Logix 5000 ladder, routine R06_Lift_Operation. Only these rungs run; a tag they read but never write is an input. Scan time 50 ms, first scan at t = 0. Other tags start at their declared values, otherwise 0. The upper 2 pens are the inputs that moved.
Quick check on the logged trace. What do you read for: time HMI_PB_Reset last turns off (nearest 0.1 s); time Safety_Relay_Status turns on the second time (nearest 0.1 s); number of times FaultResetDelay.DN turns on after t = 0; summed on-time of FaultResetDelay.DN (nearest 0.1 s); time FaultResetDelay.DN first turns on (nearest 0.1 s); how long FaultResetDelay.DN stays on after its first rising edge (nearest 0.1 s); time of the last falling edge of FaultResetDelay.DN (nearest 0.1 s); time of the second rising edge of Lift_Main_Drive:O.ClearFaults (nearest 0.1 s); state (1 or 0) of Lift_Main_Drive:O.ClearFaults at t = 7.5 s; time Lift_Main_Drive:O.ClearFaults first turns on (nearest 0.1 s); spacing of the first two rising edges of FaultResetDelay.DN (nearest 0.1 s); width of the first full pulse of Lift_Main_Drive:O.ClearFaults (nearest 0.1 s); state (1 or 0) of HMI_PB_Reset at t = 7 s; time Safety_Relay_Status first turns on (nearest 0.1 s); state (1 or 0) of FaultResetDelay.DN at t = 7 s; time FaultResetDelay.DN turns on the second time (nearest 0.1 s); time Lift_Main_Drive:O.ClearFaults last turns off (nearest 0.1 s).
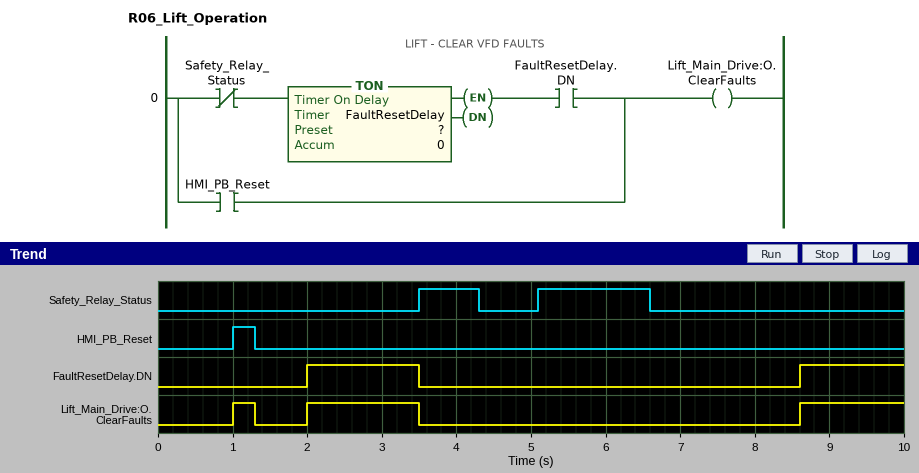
1.3 s
5.1 s
2
2.9 s
2.0 s
1.5 s
3.5 s
2.0 s
0
1.0 s
6.6 s
0.3 s
0
3.5 s
0
8.6 s
3.5 s
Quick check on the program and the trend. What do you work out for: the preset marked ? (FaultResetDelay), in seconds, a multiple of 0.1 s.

2.0 s
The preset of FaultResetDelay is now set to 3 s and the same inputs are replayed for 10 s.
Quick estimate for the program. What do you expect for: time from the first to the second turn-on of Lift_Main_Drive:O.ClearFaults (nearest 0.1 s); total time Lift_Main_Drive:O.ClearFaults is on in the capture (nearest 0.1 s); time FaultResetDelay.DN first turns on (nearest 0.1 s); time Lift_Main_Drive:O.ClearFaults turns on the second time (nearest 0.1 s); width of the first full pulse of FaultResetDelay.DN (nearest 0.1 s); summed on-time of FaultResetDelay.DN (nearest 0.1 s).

2.0 s
1.2 s
3.0 s
3.0 s
0.5 s
0.9 s
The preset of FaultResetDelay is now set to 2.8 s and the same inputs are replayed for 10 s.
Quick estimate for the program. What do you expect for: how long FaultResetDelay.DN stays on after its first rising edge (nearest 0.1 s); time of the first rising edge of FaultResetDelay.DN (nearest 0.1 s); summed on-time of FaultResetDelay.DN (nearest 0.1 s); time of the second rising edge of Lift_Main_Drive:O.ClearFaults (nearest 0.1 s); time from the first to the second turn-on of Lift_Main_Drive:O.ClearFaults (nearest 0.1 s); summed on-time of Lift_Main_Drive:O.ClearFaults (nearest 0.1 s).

0.7 s
2.8 s
1.3 s
2.8 s
1.8 s
1.6 s
